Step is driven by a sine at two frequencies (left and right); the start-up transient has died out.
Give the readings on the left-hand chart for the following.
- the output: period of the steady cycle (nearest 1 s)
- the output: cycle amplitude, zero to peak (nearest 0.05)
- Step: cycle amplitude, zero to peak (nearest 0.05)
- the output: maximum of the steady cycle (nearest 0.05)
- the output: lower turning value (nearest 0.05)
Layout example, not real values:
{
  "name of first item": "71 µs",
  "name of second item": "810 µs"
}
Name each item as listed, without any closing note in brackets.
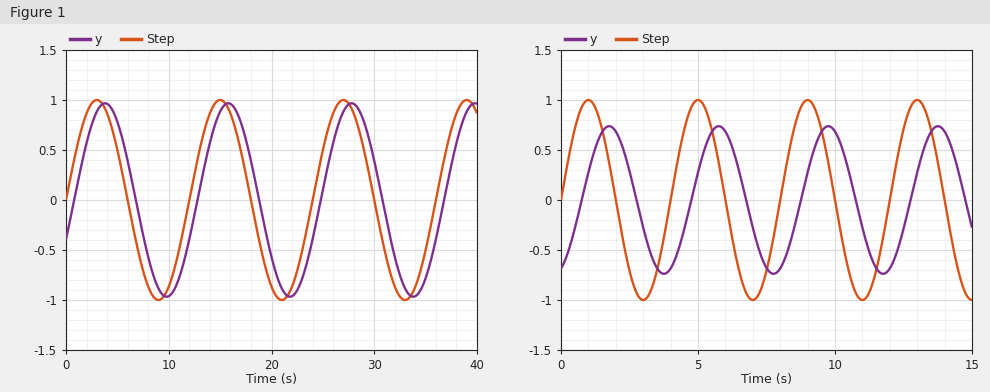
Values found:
{
  "the output: period of the steady cycle": "12 s",
  "the output: cycle amplitude, zero to peak": "0.95",
  "Step: cycle amplitude, zero to peak": "1.00",
  "the output: maximum of the steady cycle": "0.95",
  "the output: lower turning value": "-0.95"
}
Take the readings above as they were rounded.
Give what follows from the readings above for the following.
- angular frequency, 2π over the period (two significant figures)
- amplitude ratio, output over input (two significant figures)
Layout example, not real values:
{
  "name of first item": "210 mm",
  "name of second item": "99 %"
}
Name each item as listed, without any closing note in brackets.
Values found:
{
  "angular frequency, 2π over the period": "0.52 rad/s",
  "amplitude ratio, output over input": "0.95"
}
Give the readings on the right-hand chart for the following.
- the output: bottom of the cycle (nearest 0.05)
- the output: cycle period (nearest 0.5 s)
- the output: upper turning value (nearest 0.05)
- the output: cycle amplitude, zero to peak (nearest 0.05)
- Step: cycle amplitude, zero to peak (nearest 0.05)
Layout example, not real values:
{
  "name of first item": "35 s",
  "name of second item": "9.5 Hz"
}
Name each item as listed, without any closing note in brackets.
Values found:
{
  "the output: bottom of the cycle": "-0.75",
  "the output: cycle period": "4.0 s",
  "the output: upper turning value": "0.75",
  "the output: cycle amplitude, zero to peak": "0.75",
  "Step: cycle amplitude, zero to peak": "1.00"
}
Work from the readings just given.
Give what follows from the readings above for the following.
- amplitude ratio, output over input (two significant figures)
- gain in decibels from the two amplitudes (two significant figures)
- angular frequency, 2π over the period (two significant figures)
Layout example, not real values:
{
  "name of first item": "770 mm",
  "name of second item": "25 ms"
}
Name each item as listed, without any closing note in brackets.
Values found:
{
  "amplitude ratio, output over input": "0.75",
  "gain in decibels from the two amplitudes": "-2.5 dB",
  "angular frequency, 2π over the period": "1.6 rad/s"
}
